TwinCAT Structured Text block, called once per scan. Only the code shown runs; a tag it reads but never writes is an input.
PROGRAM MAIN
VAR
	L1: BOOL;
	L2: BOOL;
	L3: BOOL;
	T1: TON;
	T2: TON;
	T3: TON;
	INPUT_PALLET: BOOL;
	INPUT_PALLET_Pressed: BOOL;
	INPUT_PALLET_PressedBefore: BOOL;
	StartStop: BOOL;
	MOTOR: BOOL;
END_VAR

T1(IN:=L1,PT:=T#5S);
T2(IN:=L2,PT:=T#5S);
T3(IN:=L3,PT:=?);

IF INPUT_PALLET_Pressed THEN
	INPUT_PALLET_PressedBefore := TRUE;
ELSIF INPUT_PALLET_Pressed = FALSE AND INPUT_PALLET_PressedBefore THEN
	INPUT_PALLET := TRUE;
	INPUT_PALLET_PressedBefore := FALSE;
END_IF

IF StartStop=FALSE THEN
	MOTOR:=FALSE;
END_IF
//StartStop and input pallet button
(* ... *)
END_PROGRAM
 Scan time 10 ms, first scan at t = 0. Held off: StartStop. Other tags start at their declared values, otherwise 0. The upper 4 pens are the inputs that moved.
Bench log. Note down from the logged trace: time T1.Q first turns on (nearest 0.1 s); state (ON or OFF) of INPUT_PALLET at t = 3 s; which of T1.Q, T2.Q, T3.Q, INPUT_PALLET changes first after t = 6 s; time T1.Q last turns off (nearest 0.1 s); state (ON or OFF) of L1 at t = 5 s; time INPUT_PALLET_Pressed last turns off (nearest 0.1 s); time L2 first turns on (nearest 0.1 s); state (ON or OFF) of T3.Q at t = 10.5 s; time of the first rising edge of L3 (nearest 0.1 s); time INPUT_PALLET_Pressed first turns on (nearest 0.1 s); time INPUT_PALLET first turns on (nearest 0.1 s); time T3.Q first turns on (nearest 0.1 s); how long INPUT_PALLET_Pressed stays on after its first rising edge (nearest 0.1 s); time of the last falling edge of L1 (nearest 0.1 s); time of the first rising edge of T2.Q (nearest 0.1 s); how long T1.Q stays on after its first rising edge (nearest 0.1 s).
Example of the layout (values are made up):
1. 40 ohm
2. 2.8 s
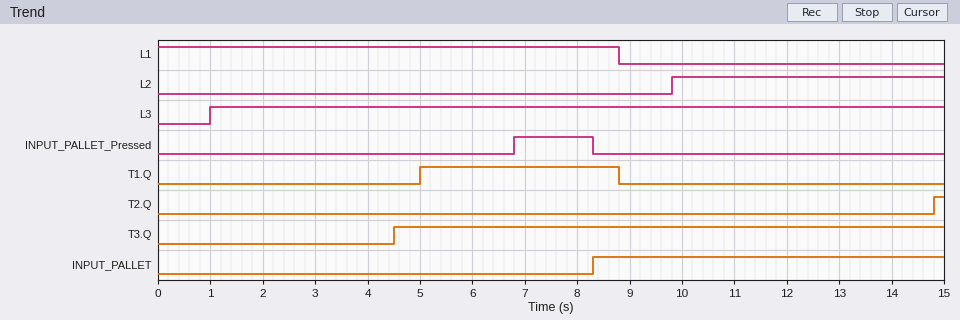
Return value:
1. 5.0 s
2. OFF
3. INPUT_PALLET
4. 8.8 s
5. ON
6. 8.3 s
7. 9.8 s
8. ON
9. 1.0 s
10. 6.8 s
11. 8.3 s
12. 4.5 s
13. 1.5 s
14. 8.8 s
15. 14.8 s
16. 3.8 s
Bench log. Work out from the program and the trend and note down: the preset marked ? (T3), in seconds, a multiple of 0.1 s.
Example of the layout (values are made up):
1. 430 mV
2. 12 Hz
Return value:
1. 3.5 s
